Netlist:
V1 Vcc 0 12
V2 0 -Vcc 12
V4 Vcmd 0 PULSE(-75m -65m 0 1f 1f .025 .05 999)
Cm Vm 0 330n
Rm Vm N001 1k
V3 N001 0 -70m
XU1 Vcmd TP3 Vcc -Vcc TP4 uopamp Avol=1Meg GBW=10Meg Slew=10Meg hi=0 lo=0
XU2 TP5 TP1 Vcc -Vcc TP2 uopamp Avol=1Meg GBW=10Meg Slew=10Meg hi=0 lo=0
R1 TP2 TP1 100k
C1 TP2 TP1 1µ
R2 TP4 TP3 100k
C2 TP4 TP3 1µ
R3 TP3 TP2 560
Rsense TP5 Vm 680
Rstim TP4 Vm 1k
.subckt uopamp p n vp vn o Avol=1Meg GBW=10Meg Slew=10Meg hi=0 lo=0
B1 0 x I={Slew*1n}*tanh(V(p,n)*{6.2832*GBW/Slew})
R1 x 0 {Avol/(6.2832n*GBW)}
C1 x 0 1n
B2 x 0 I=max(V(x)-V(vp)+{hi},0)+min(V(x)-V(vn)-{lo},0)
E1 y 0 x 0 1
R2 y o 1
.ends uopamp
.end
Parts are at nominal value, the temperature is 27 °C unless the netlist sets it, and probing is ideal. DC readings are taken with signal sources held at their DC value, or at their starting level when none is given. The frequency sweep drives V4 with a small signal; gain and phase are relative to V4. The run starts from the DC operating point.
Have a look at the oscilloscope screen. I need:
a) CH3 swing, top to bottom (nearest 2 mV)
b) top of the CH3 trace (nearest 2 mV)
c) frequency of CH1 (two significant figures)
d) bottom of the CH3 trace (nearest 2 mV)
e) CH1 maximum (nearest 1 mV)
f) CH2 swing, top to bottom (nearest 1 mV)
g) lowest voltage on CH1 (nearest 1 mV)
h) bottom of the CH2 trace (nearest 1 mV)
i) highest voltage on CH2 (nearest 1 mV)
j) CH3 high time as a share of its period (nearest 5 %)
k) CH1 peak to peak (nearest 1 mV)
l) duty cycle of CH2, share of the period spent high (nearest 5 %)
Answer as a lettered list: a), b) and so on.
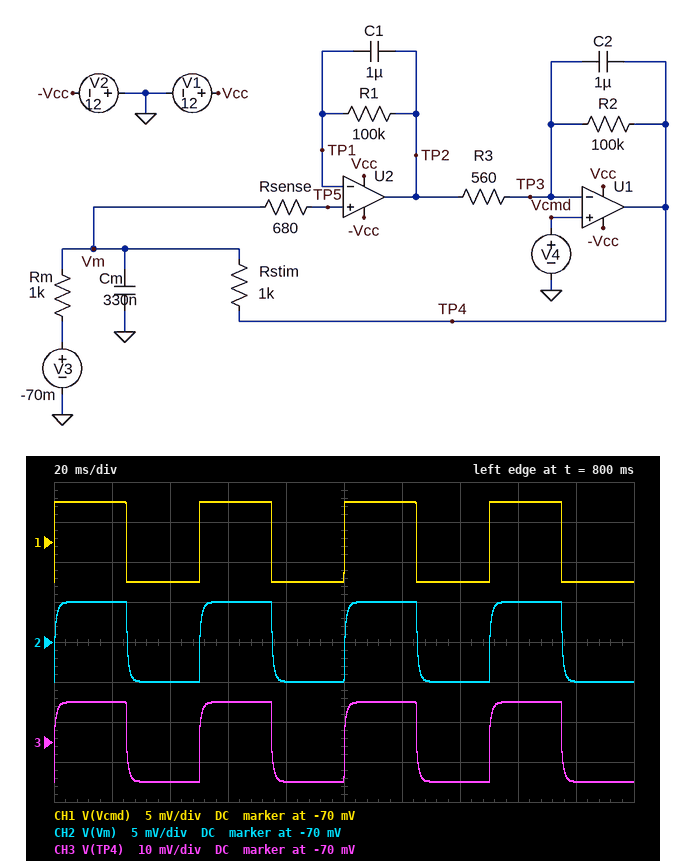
a) 20 mV
b) -60 mV
c) 20 Hz
d) -80 mV
e) -65 mV
f) 10 mV
g) -75 mV
h) -75 mV
i) -65 mV
j) 50 %
k) 10 mV
l) 50 %
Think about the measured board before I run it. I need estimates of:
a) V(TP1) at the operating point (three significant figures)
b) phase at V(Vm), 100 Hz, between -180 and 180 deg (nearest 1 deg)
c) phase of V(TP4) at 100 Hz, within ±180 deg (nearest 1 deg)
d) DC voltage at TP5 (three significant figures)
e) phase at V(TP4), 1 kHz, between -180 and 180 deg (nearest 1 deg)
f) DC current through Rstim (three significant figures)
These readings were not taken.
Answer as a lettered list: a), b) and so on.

a) -75.0 mV
b) -18 deg
c) -12 deg
d) -75.0 mV
e) -12 deg
f) 4.97 µA
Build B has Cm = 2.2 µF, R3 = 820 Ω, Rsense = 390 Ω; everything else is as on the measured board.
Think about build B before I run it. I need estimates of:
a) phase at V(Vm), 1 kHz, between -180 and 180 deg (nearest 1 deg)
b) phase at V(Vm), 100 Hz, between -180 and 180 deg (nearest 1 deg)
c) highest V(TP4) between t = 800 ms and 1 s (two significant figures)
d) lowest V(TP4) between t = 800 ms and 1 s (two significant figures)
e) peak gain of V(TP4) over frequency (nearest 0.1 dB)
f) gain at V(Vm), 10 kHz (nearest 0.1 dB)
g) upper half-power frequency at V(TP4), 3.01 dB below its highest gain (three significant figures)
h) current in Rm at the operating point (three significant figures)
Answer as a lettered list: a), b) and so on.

a) -93 deg
b) -47 deg
c) -56 mV
d) -84 mV
e) 8.1 dB
f) -42.8 dB
g) 197 Hz
h) 4.96 µA
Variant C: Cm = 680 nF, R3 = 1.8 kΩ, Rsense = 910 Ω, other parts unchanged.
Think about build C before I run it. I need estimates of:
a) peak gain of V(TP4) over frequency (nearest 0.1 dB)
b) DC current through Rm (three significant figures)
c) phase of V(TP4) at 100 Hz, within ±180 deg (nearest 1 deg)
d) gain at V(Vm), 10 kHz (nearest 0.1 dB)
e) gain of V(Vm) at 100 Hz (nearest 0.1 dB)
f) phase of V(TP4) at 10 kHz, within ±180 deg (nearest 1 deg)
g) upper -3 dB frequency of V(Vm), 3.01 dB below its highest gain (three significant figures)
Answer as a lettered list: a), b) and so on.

a) 5.9 dB
b) 4.91 µA
c) -16 deg
d) -32.6 dB
e) -3.7 dB
f) -1 deg
g) 80.6 Hz
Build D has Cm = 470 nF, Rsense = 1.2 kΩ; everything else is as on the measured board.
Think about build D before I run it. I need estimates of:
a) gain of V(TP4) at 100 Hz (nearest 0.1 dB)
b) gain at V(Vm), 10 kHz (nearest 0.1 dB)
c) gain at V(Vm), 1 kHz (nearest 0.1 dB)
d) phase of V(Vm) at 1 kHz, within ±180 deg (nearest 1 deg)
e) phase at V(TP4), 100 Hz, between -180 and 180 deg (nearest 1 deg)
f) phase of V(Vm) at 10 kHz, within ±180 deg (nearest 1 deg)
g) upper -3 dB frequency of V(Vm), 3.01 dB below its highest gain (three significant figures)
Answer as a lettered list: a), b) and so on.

a) 5.5 dB
b) -29.4 dB
c) -10.1 dB
d) -69 deg
e) -10 deg
f) -88 deg
g) 286 Hz
